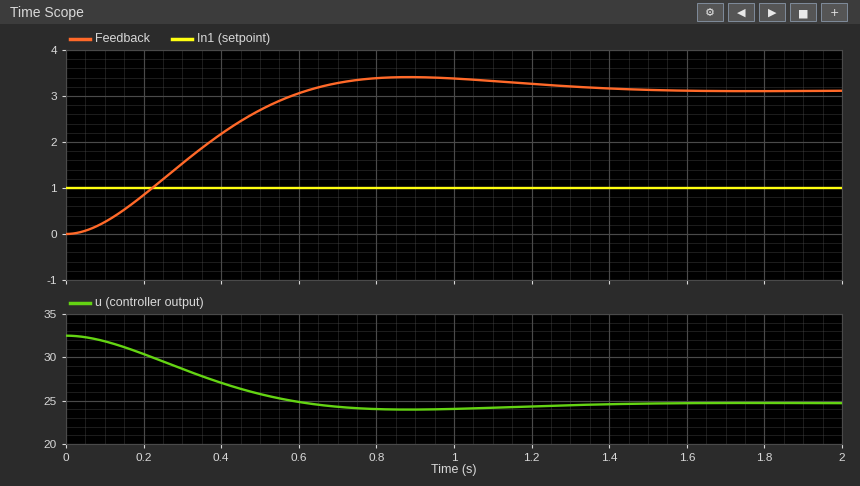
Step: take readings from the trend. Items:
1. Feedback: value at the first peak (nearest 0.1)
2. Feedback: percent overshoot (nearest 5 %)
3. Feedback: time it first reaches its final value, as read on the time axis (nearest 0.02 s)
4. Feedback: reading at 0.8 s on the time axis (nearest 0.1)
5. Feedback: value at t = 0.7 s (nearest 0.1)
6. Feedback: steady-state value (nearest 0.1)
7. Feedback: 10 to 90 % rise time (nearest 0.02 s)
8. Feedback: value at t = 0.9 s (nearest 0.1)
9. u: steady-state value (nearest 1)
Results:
3.4
10 %
0.62 s
3.4
3.3
3.1
0.42 s
3.4
25
